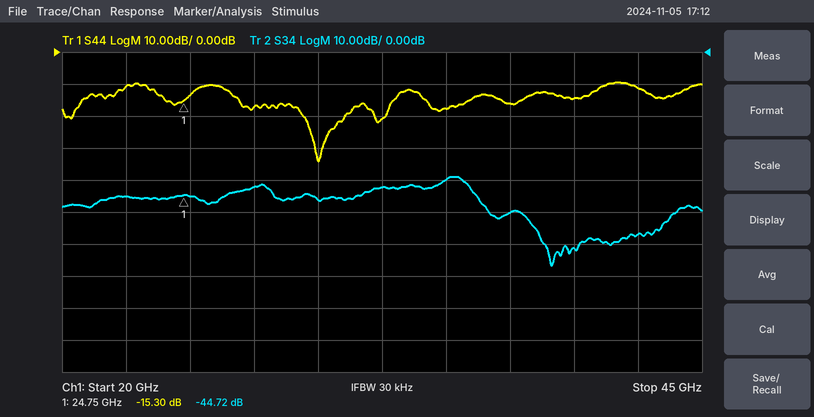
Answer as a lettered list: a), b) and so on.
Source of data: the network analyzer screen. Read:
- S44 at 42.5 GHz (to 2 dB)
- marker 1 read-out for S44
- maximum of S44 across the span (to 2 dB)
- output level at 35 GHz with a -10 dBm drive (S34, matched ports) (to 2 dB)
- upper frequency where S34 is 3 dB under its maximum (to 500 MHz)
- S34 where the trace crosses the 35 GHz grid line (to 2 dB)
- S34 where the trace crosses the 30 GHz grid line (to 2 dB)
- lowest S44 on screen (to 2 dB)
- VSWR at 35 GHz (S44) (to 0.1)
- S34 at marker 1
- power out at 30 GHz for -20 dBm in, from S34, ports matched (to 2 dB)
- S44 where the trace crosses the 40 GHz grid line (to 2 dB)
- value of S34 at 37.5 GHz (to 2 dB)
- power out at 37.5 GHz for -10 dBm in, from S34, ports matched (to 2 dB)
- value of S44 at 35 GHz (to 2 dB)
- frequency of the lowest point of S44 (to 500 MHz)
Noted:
a) -12 dB
b) -15.30 dB
c) -10 dB
d) -50 dBm
e) 36.0 GHz
f) -40 dB
g) -46 dB
h) -34 dB
i) 1.3
j) -44.72 dB
k) -66 dBm
l) -14 dB
m) -50 dB
n) -60 dBm
o) -18 dB
p) 30.0 GHz
